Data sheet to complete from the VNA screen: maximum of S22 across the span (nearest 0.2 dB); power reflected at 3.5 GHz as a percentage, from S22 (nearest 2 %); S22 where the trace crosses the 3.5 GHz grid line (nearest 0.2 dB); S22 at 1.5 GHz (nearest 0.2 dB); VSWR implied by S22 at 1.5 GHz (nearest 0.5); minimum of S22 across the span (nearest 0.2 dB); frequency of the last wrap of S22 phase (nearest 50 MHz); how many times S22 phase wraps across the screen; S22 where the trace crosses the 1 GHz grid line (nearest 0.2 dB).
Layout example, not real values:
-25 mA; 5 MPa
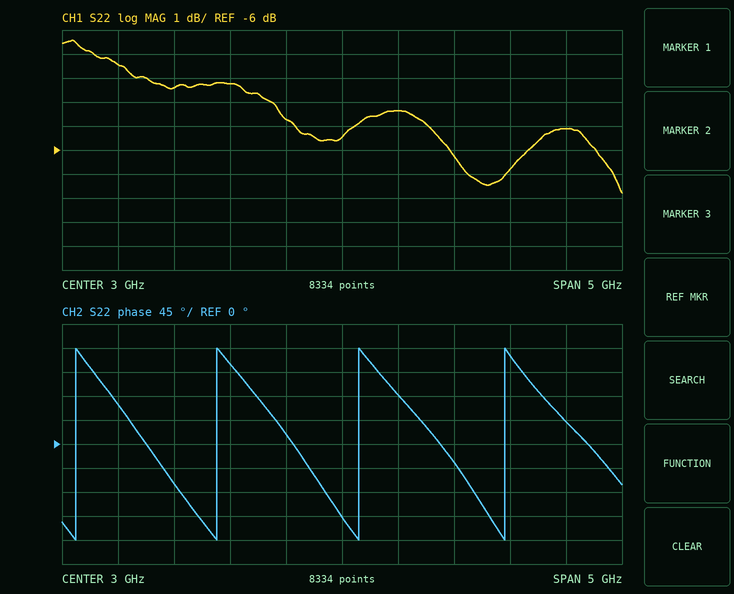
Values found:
-1.4 dB; 36 %; -4.4 dB; -3.4 dB; 5.0; -7.8 dB; 4.45 GHz; 4; -2.4 dB
